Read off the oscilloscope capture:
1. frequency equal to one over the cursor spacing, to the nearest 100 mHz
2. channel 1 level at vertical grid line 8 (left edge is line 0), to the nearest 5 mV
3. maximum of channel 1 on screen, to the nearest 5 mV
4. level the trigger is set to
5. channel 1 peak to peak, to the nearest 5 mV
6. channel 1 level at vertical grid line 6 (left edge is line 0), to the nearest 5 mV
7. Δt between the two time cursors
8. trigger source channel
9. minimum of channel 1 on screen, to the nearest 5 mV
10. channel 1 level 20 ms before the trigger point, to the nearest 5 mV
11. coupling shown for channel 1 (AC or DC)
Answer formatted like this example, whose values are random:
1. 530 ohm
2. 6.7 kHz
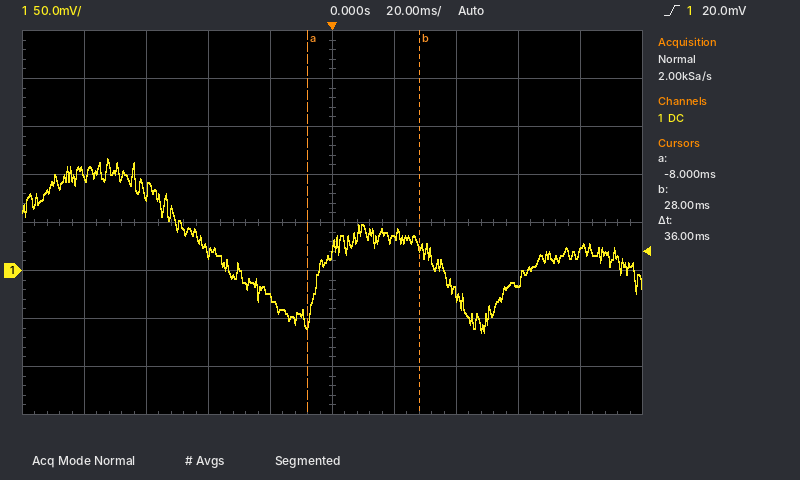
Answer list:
1. 27.8 Hz
2. -10 mV
3. 115 mV
4. 20.0 mV
5. 180 mV
6. 35 mV
7. 36 ms
8. channel 1
9. -65 mV
10. -30 mV
11. DC
